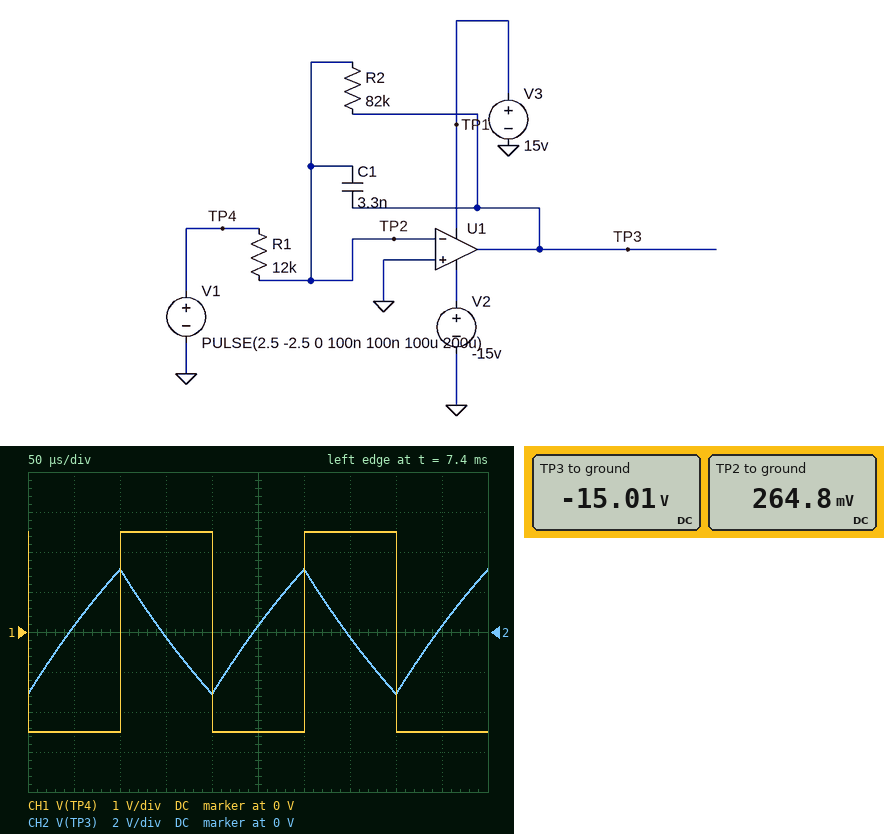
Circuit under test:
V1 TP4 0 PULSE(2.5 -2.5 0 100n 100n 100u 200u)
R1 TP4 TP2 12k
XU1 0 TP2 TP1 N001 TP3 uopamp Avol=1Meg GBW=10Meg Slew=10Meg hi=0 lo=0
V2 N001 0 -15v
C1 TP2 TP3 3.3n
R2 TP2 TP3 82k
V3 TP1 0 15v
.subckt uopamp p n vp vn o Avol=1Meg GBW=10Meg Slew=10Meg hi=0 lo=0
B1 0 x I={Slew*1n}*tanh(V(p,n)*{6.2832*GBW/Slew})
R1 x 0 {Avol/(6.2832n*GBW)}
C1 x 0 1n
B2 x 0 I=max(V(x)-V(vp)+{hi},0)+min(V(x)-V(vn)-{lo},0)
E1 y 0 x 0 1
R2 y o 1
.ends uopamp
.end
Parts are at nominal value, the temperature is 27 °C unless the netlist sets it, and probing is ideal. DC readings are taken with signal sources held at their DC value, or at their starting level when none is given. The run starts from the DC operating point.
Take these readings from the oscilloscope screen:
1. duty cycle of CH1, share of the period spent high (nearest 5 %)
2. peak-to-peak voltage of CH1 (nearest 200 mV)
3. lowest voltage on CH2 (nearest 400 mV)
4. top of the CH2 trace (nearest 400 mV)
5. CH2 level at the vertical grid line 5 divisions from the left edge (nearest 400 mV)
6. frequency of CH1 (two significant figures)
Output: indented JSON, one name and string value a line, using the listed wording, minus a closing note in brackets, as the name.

{
  "duty cycle of CH1, share of the period spent high": "50 %",
  "peak-to-peak voltage of CH1": "5.0 V",
  "lowest voltage on CH2": "-3.2 V",
  "top of the CH2 trace": "3.2 V",
  "CH2 level at the vertical grid line 5 divisions from the left edge": "400 mV",
  "frequency of CH1": "5.0 kHz"
}
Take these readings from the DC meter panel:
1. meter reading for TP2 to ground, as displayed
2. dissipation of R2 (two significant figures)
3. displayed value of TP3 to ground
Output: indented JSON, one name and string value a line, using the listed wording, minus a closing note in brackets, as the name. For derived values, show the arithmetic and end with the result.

{
  "meter reading for TP2 to ground, as displayed": "264.8 mV",
  "dissipation of R2": "(264.8 mV - (-15.01 V))^2 / 82 kΩ = 2.8 mW",
  "displayed value of TP3 to ground": "-15.01 V"
}
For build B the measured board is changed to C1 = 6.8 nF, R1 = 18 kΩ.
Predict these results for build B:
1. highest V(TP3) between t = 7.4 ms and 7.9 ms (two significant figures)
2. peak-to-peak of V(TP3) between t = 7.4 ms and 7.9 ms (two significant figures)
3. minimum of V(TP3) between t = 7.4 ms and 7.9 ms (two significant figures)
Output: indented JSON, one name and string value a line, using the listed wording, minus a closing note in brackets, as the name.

{
  "highest V(TP3) between t = 7.4 ms and 7.9 ms": "1.0 V",
  "peak-to-peak of V(TP3) between t = 7.4 ms and 7.9 ms": "2.0 V",
  "minimum of V(TP3) between t = 7.4 ms and 7.9 ms": "-1.0 V"
}
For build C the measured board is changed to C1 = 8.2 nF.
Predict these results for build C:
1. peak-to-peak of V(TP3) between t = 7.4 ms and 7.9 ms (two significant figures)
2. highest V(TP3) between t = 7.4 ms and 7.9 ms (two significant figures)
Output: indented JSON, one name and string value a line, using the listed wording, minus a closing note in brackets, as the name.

{
  "peak-to-peak of V(TP3) between t = 7.4 ms and 7.9 ms": "2.5 V",
  "highest V(TP3) between t = 7.4 ms and 7.9 ms": "1.3 V"
}
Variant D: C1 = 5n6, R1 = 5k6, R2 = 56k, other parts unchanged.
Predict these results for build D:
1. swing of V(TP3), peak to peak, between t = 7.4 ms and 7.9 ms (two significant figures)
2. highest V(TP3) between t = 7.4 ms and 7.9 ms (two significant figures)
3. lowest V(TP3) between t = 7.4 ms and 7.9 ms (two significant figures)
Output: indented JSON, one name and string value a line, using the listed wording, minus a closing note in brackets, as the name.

{
  "swing of V(TP3), peak to peak, between t = 7.4 ms and 7.9 ms": "7.9 V",
  "highest V(TP3) between t = 7.4 ms and 7.9 ms": "4.0 V",
  "lowest V(TP3) between t = 7.4 ms and 7.9 ms": "-3.9 V"
}
